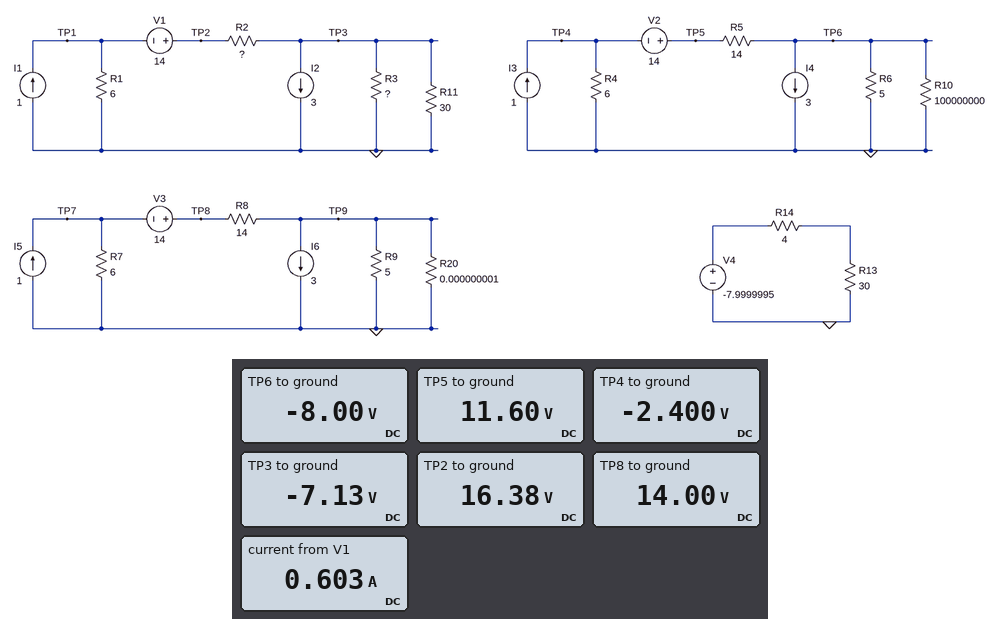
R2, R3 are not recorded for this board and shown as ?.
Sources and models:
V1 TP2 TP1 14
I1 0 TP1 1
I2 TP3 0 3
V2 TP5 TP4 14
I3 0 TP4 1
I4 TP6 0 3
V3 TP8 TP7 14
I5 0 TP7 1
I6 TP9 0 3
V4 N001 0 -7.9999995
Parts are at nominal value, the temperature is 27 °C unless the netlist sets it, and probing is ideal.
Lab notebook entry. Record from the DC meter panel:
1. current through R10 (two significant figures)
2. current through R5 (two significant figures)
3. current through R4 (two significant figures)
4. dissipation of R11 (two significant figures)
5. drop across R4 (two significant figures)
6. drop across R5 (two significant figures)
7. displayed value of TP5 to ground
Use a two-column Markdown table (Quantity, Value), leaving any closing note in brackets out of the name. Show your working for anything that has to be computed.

| Quantity | Value |
|---|---|
| current through R10 | (0 V - (-8 V)) / 100 MΩ = 80 nA |
| current through R5 | (11.6 V - (-8 V)) / 14 Ω = 1.4 A |
| current through R4 | (0 V - (-2.4 V)) / 6 Ω = 400 mA |
| dissipation of R11 | (0 V - (-7.13 V))^2 / 30 Ω = 1.7 W |
| drop across R4 | 0 V - (-2.4 V) = 2.4 V |
| drop across R5 | 11.6 V - (-8 V) = 20 V |
| displayed value of TP5 to ground | 11.60 V |
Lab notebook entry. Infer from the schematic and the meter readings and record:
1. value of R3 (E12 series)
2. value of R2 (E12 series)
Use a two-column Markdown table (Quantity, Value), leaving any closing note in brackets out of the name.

| Quantity | Value |
|---|---|
| value of R3 | 3.3 Ω |
| value of R2 | 39 Ω |
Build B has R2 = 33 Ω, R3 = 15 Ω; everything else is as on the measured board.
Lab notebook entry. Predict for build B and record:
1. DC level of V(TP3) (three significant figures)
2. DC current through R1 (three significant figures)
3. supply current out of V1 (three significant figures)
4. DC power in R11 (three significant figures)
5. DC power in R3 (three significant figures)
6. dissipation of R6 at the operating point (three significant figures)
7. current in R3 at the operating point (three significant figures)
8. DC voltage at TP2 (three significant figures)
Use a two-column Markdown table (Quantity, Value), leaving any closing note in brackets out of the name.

| Quantity | Value |
|---|---|
| DC level of V(TP3) | -19.8 V |
| DC current through R1 | 20.4 mA |
| supply current out of V1 | 1.02 A |
| DC power in R11 | 13.1 W |
| DC power in R3 | 26.1 W |
| dissipation of R6 at the operating point | 12.8 W |
| current in R3 at the operating point | 1.32 A |
| DC voltage at TP2 | 13.9 V |
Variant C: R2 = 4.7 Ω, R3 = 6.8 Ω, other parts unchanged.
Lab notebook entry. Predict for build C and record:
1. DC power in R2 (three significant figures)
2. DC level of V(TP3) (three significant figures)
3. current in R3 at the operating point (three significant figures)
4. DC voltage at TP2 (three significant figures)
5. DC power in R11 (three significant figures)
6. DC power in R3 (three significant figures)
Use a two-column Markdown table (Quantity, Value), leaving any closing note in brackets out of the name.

| Quantity | Value |
|---|---|
| DC power in R2 | 23.9 W |
| DC level of V(TP3) | -4.13 V |
| current in R3 at the operating point | 607 mA |
| DC voltage at TP2 | 6.47 V |
| DC power in R11 | 568 mW |
| DC power in R3 | 2.51 W |
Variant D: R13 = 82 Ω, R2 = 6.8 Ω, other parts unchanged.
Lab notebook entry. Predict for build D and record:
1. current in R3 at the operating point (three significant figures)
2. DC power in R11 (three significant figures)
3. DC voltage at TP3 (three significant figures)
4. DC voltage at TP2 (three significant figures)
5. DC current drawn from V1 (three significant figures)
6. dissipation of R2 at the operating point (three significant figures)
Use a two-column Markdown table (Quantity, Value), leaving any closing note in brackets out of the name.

| Quantity | Value |
|---|---|
| current in R3 at the operating point | 1.05 A |
| DC power in R11 | 401 mW |
| DC voltage at TP3 | -3.47 V |
| DC voltage at TP2 | 9.00 V |
| DC current drawn from V1 | 1.83 A |
| dissipation of R2 at the operating point | 22.9 W |
